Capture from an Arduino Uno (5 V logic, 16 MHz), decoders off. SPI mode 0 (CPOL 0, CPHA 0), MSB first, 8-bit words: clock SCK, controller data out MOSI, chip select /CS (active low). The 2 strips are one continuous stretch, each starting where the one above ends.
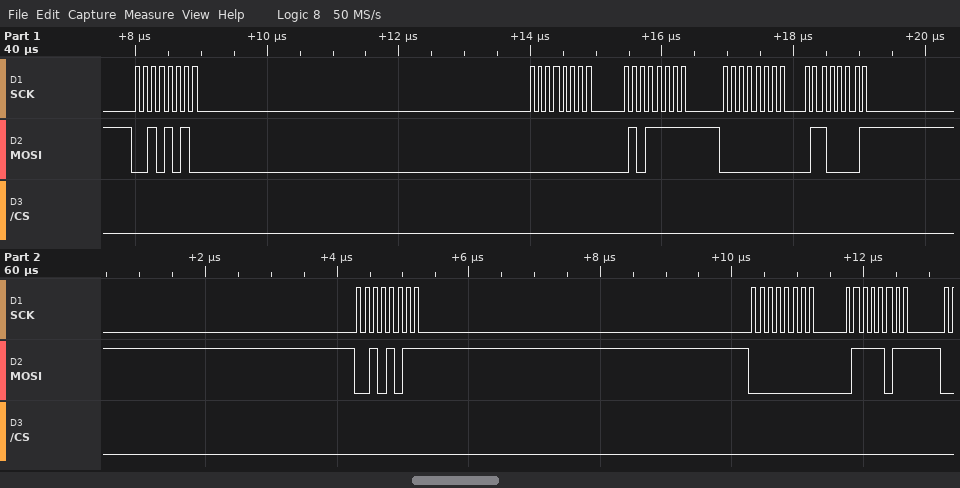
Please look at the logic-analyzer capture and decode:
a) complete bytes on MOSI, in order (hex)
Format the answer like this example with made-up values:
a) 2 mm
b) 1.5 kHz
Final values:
a) 2A 00 5F 00 61 2B 00 7B
